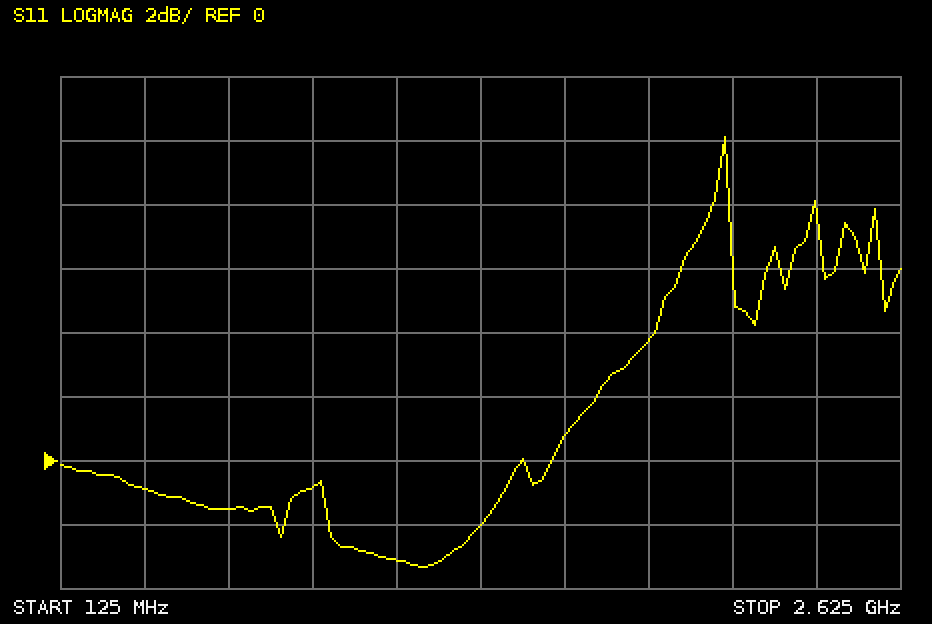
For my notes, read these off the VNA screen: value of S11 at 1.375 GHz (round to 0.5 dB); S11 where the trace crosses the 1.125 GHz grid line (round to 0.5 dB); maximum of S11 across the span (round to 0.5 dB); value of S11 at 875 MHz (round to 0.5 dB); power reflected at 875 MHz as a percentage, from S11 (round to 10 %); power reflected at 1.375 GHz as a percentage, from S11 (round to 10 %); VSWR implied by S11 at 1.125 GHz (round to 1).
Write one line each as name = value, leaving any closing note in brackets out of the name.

value of S11 at 1.375 GHz = -2.0 dB
S11 where the trace crosses the 1.125 GHz grid line = -3.0 dB
maximum of S11 across the span = 10.0 dB
value of S11 at 875 MHz = -1.0 dB
power reflected at 875 MHz as a percentage, from S11 = 80 %
power reflected at 1.375 GHz as a percentage, from S11 = 60 %
VSWR implied by S11 at 1.125 GHz = 6
